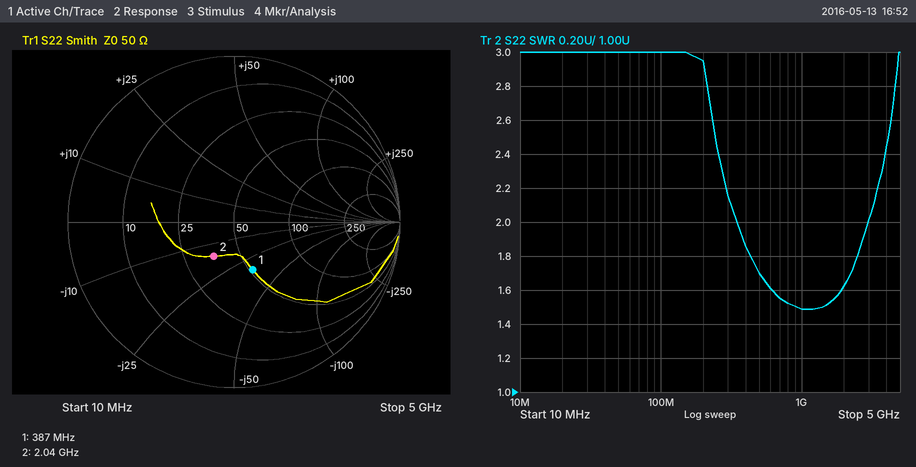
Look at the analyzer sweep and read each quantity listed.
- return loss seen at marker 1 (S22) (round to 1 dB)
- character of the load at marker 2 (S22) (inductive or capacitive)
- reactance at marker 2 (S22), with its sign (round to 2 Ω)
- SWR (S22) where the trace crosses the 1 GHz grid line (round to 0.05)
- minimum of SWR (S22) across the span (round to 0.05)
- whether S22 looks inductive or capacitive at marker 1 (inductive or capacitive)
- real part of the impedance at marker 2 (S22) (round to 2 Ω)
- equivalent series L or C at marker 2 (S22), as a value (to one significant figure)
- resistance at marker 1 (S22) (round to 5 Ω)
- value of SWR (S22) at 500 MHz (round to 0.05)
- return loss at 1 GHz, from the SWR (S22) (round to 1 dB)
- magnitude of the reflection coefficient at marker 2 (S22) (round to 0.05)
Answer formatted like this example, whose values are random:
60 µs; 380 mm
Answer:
10 dB; capacitive; -16 Ω; 1.50; 1.50; capacitive; 36 Ω; 5 pF; 50 Ω; 1.70; 14 dB; 0.25
